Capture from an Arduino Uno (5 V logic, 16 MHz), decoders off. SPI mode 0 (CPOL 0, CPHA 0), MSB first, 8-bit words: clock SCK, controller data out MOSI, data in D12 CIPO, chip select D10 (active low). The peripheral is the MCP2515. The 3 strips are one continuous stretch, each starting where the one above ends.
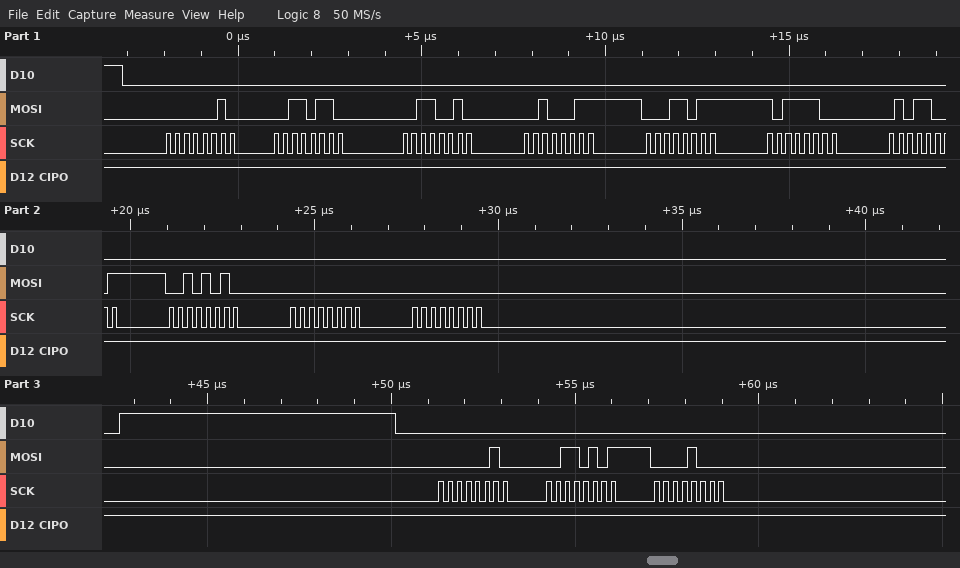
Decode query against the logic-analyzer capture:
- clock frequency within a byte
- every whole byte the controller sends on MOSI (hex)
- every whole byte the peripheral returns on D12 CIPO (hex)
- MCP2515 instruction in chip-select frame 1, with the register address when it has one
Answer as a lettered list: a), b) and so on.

a) 4 MHz
b) 0x02 0x36 0x32 0x23 0x1B 0xBC 0x59 0x2A 0x00 0x00 0x02 0x35 0x08
c) 0xFF 0xFF 0xFF 0xFF 0xFF 0xFF 0xFF 0xFF 0xFF 0xFF 0xFF 0xFF 0xFF
d) WRITE 0x36
